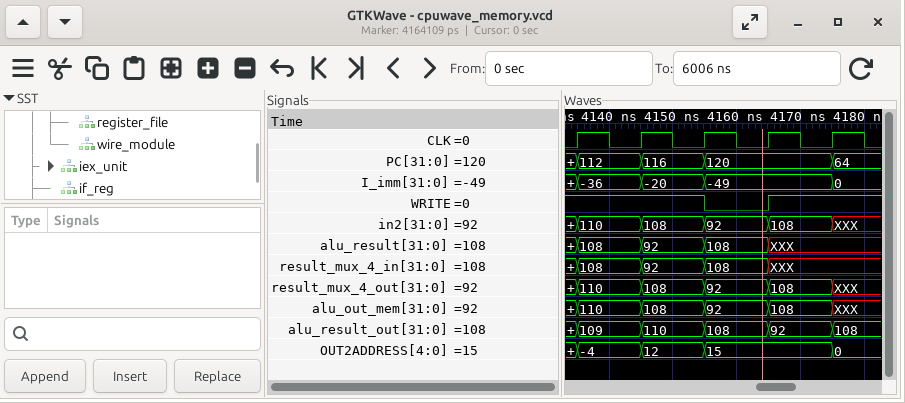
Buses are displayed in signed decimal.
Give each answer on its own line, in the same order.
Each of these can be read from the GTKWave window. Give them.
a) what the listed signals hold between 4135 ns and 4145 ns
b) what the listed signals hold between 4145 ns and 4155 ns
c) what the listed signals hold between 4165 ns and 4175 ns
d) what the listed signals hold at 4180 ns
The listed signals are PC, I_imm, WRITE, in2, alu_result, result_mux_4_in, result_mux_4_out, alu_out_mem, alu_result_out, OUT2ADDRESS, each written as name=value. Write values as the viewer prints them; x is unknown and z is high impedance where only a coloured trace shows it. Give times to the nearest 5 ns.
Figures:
PC=112, I_imm=-36, WRITE=1, in2=110, alu_result=108, result_mux_4_in=108, result_mux_4_out=110, alu_out_mem=110, alu_result_out=109, OUT2ADDRESS=-4
PC=116, I_imm=-20, WRITE=1, in2=108, alu_result=92, result_mux_4_in=92, result_mux_4_out=108, alu_out_mem=108, alu_result_out=110, OUT2ADDRESS=12
PC=120, I_imm=-49, WRITE=1, in2=108, alu_result=XXX, result_mux_4_in=XXX, result_mux_4_out=108, alu_out_mem=108, alu_result_out=92, OUT2ADDRESS=15
PC=64, I_imm=0, WRITE=1, in2=XXX, alu_result=XXX, result_mux_4_in=XXX, result_mux_4_out=XXX, alu_out_mem=XXX, alu_result_out=108, OUT2ADDRESS=0
